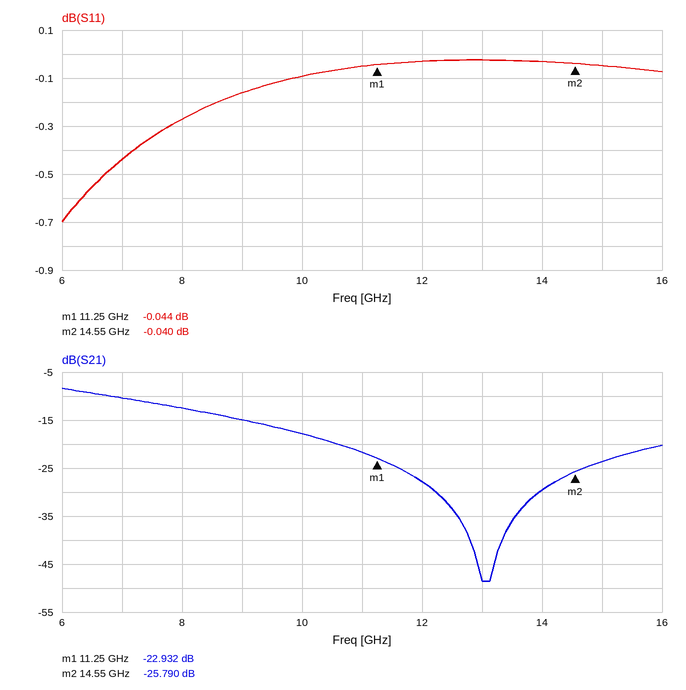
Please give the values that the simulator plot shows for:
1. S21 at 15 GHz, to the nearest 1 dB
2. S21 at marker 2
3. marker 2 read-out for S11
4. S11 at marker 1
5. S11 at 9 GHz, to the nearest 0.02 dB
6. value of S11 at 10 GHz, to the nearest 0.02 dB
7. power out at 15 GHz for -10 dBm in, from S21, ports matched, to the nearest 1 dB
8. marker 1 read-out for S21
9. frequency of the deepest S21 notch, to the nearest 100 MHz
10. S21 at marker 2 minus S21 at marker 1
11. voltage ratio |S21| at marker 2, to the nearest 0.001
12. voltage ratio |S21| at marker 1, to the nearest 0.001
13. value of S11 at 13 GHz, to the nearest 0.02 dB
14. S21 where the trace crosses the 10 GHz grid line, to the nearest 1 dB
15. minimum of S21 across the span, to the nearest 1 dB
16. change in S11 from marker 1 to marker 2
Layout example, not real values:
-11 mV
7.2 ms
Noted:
-24 dB
-25.790 dB
-0.040 dB
-0.044 dB
-0.16 dB
-0.10 dB
-34 dBm
-22.932 dB
13.0 GHz
-2.858 dB
0.051
0.071
-0.02 dB
-18 dB
-49 dB
0.004 dB
